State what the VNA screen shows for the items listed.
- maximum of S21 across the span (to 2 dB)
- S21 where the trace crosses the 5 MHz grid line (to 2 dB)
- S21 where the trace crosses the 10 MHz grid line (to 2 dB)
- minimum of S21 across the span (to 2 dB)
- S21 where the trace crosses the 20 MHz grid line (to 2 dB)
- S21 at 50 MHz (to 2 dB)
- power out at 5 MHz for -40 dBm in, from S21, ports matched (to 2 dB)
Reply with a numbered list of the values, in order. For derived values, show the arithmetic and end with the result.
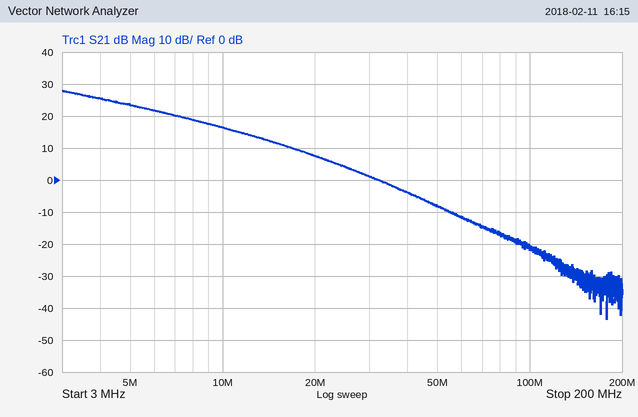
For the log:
1. 28 dB
2. 24 dB
3. 16 dB
4. -44 dB
5. 8 dB
6. -8 dB
7. -40 dBm + (24 dB) = -16 dBm
